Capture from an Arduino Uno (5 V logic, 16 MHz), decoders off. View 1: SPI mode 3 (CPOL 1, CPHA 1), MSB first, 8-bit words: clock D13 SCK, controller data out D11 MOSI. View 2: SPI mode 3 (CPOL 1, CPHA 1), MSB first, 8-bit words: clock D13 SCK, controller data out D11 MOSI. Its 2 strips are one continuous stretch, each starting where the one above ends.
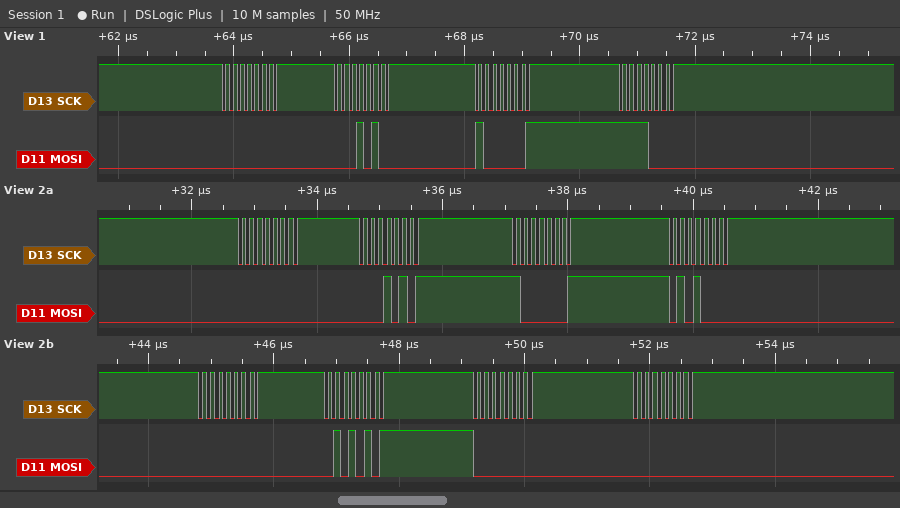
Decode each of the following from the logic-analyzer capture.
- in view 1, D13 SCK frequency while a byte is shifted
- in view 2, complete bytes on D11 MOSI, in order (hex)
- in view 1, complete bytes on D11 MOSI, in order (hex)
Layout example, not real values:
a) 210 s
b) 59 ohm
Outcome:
a) 8 MHz
b) 00 15 81 50 00 55 00 00
c) 00 14 81 F0
